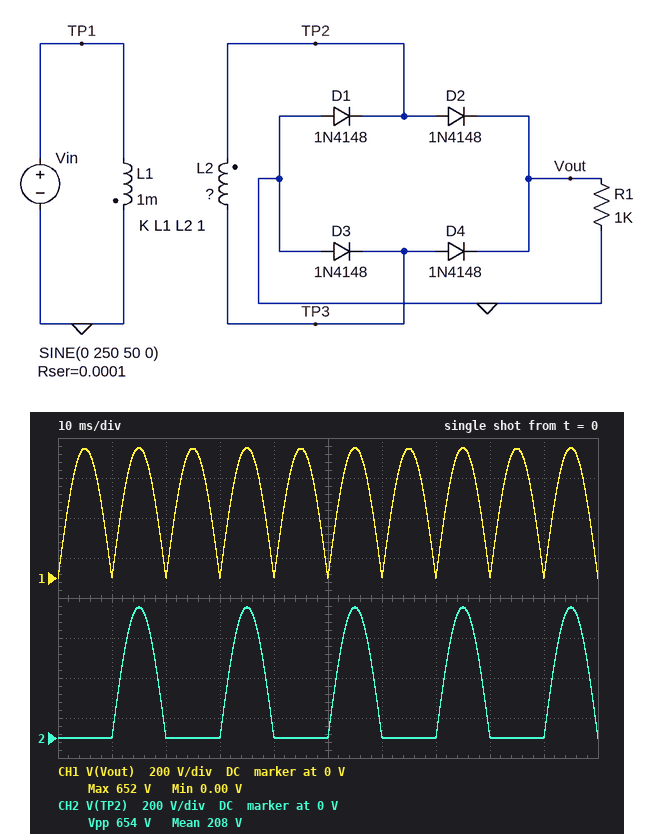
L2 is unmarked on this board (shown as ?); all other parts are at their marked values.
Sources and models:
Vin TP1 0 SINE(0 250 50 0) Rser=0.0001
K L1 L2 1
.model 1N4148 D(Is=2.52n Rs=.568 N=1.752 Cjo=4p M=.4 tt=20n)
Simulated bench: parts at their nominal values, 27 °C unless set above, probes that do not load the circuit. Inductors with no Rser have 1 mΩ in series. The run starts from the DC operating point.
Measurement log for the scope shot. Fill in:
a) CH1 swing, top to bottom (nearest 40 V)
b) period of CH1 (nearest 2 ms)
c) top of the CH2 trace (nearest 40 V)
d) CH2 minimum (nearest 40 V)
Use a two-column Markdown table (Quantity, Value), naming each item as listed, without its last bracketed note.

| Quantity | Value |
|---|---|
| CH1 swing, top to bottom | 640 V |
| period of CH1 | 10 ms |
| top of the CH2 trace | 640 V |
| CH2 minimum | 0 V |
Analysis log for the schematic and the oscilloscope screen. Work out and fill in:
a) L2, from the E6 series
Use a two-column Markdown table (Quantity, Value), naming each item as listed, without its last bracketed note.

| Quantity | Value |
|---|---|
| L2, from the E6 series | 6.8 mH |
